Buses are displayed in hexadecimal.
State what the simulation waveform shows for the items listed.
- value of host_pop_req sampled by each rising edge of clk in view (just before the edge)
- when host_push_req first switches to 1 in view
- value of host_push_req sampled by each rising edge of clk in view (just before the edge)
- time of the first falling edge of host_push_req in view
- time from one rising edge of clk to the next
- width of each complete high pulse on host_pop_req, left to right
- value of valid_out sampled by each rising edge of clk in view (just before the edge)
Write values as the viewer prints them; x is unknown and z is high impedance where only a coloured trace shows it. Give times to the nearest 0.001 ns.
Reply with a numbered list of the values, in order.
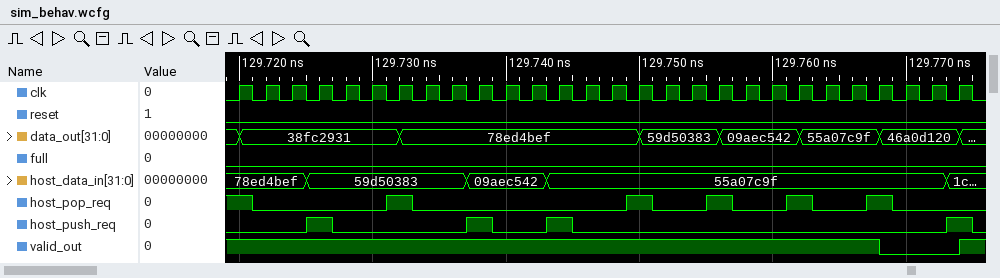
1. 1 0 0 0 0 0 1 0 0 0 0 0 0 0 0 1 0 0 1 0 0 1 0 0 1 0 0 0
2. 129.725 ns
3. 0 0 0 1 0 0 0 0 0 1 0 0 1 0 0 0 0 0 0 0 0 0 0 0 0 0 0 1
4. 129.727 ns
5. 0.002 ns
6. 0.002 ns, 0.002 ns, 0.002 ns, 0.002 ns, 0.002 ns
7. 1 1 1 1 1 1 1 1 1 1 1 1 1 1 1 1 1 1 1 1 1 1 1 1 1 0 0 0
